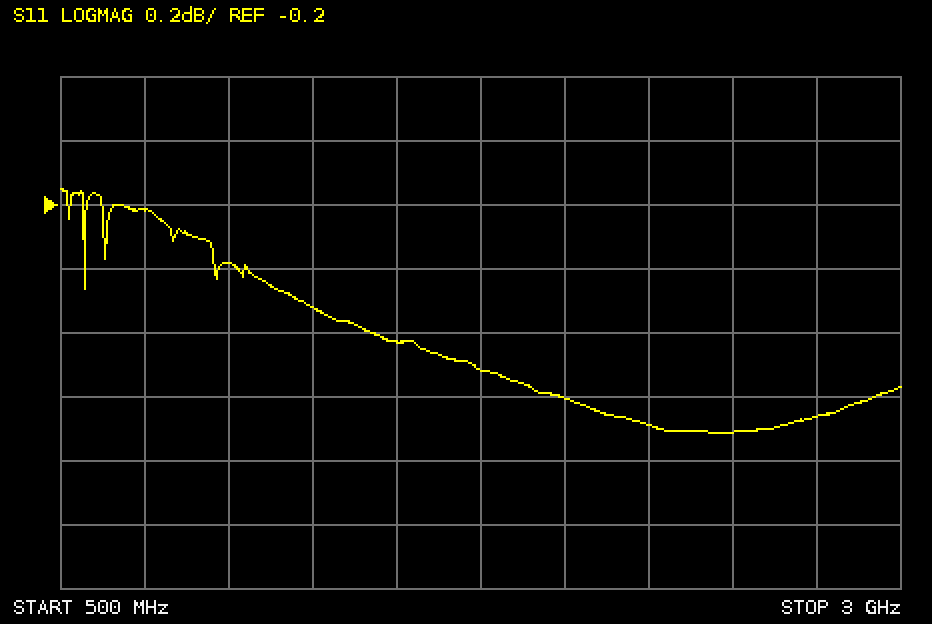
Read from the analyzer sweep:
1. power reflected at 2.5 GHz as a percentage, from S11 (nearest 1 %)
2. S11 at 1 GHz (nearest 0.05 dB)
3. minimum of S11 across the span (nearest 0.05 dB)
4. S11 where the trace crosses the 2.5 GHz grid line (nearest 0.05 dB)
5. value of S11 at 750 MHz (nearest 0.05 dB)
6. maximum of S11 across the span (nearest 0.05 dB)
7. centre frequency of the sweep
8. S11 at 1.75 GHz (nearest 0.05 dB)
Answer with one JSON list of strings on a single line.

["81 %", "-0.40 dB", "-0.90 dB", "-0.90 dB", "-0.20 dB", "-0.15 dB", "1.75 GHz", "-0.70 dB"]
